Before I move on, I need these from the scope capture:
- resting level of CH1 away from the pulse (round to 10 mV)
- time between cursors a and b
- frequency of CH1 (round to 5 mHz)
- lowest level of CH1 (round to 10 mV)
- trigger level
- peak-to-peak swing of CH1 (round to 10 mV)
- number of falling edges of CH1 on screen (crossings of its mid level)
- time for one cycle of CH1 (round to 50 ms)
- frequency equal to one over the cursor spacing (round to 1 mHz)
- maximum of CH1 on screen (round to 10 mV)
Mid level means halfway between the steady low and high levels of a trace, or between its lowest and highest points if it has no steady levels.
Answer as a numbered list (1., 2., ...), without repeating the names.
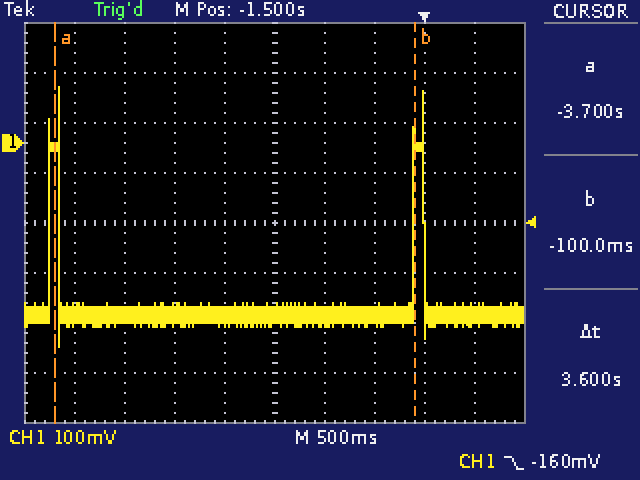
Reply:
1. -340 mV
2. 3.6 s
3. 275 mHz
4. -410 mV
5. -160 mV
6. 520 mV
7. 2
8. 3.65 s
9. 278 mHz
10. 110 mV
